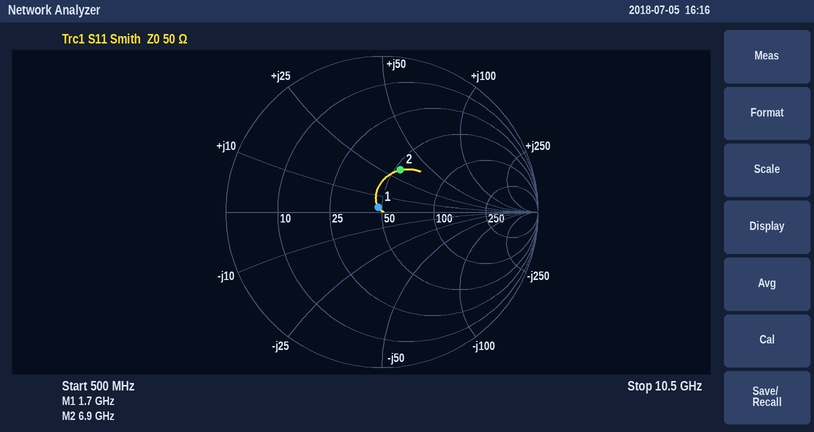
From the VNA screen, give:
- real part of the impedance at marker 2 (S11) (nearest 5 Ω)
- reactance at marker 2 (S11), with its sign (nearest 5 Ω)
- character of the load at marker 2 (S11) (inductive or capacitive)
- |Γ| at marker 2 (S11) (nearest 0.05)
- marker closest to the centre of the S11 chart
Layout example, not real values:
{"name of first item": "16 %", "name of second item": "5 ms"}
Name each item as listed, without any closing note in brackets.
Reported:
{"real part of the impedance at marker 2 (S11)": "55 Ω", "reactance at marker 2 (S11), with its sign": "+30 Ω", "character of the load at marker 2 (S11)": "inductive", "|Γ| at marker 2 (S11)": "0.30", "marker closest to the centre of the S11 chart": "marker 1"}
